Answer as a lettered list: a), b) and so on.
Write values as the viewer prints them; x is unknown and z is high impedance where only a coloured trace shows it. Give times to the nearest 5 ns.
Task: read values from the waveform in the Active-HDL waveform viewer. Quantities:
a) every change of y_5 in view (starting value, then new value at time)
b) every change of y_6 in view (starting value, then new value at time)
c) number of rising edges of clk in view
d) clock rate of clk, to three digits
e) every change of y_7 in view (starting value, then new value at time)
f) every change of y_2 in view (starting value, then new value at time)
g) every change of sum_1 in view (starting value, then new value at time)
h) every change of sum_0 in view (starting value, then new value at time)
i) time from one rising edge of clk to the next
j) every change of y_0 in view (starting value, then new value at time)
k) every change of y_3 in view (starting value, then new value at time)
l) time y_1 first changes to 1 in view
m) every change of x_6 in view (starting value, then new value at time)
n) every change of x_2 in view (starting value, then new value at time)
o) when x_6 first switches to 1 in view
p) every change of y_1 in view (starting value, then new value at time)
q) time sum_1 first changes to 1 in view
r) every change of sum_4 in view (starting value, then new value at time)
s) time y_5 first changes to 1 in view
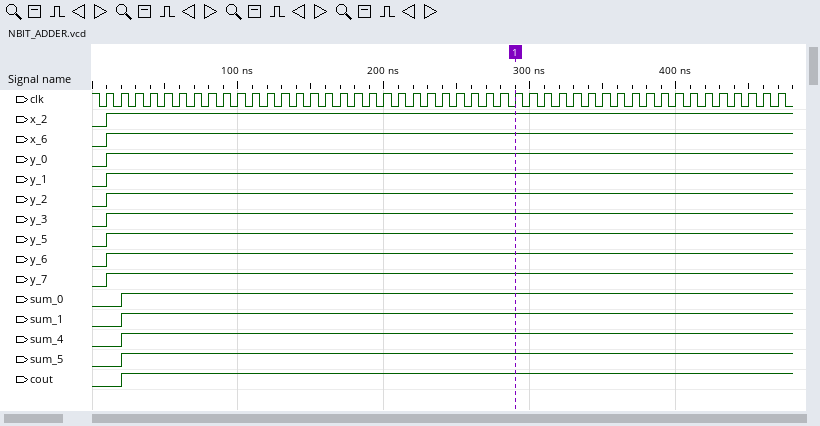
a) 0, 1 at 10 ns
b) 0, 1 at 10 ns
c) 47
d) 100 MHz
e) 0, 1 at 10 ns
f) 0, 1 at 10 ns
g) 0, 1 at 20 ns
h) 0, 1 at 20 ns
i) 10 ns
j) 0, 1 at 10 ns
k) 0, 1 at 10 ns
l) 10 ns
m) 0, 1 at 10 ns
n) 0, 1 at 10 ns
o) 10 ns
p) 0, 1 at 10 ns
q) 20 ns
r) 0, 1 at 20 ns
s) 10 ns
